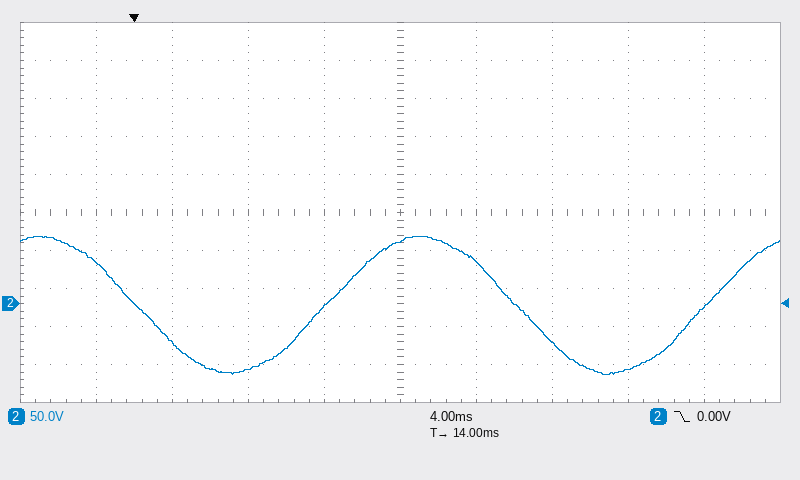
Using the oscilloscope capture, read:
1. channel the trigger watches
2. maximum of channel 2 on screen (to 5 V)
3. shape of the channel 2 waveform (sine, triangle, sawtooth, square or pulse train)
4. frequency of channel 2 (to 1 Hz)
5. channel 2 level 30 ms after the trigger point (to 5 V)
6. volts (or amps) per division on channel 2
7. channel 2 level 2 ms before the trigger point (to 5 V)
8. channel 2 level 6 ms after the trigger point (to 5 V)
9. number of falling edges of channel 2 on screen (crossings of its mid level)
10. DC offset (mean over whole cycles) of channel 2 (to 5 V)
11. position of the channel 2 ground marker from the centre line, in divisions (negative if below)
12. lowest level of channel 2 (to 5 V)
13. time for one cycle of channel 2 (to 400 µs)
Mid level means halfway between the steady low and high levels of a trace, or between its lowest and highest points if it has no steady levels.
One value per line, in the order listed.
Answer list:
channel 2
90 V
sine
50 Hz
-5 V
50 V
55 V
-85 V
2
0 V
-2.4 div
-95 V
20.0 ms
